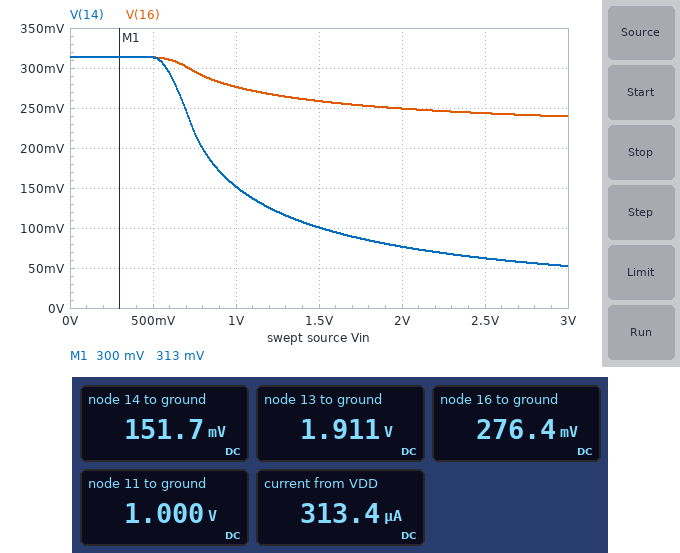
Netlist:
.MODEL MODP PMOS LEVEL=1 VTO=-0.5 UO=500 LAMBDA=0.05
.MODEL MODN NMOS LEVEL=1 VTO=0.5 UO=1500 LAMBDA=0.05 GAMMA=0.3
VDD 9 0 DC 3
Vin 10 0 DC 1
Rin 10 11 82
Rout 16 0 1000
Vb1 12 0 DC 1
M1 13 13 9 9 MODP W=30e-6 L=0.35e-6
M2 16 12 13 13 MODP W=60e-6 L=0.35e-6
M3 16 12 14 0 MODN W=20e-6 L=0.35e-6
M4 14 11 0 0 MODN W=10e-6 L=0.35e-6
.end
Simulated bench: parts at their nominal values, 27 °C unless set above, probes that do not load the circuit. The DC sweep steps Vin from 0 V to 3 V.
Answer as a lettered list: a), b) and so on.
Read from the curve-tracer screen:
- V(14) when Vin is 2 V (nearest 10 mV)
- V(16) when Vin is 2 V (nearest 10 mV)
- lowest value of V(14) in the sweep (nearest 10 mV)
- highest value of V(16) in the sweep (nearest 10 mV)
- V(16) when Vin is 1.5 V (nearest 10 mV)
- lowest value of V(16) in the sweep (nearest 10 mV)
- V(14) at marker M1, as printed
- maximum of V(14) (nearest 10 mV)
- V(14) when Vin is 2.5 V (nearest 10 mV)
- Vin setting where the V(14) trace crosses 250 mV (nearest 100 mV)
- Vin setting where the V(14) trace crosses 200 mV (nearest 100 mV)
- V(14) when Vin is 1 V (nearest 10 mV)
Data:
a) 80 mV
b) 250 mV
c) 50 mV
d) 310 mV
e) 260 mV
f) 240 mV
g) 313 mV
h) 310 mV
i) 60 mV
j) 700 mV
k) 800 mV
l) 150 mV
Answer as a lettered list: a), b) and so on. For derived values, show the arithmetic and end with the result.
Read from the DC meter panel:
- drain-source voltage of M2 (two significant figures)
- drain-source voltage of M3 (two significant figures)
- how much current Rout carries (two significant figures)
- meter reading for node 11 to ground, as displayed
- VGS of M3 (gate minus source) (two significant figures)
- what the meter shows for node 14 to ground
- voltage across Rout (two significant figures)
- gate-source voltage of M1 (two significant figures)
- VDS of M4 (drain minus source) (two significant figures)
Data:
a) 276.4 mV - 1.911 V = -1.6 V
b) 276.4 mV - 151.7 mV = 120 mV
c) (276.4 mV) / 1 kΩ = 280 µA
d) 1.000 V
e) 1 V - 151.7 mV = 850 mV
f) 151.7 mV
g) 276.4 mV = 280 mV
h) 1.911 V - 3 V = -1.1 V
i) 151.7 mV = 150 mV
